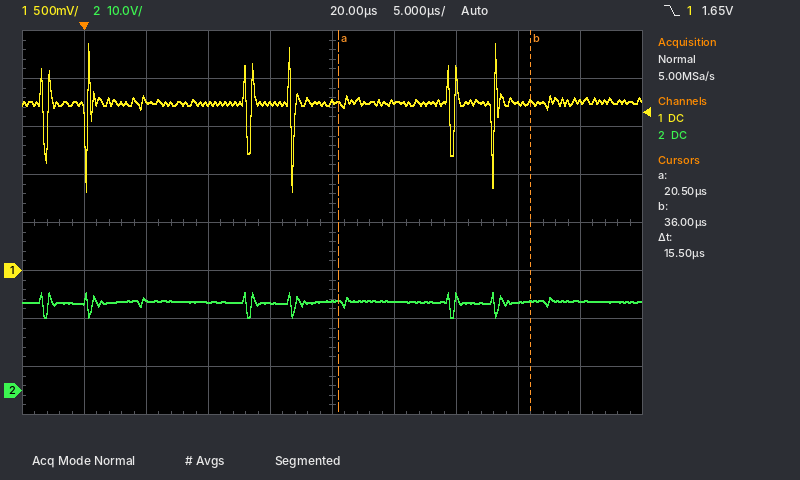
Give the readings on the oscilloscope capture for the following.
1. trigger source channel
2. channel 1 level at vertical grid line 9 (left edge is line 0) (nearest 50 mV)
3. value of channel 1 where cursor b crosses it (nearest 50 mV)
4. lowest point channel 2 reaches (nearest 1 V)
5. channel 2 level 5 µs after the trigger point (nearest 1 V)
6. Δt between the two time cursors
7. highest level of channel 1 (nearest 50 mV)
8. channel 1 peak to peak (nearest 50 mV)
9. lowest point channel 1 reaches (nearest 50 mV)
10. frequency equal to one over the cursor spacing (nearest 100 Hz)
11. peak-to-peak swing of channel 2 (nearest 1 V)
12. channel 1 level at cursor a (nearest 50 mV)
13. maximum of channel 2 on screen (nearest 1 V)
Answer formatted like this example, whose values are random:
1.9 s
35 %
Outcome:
channel 1
1.75 V
1.75 V
15 V
19 V
15.5 µs
2.35 V
1.55 V
800 mV
64.5 kHz
5 V
1.75 V
20 V
